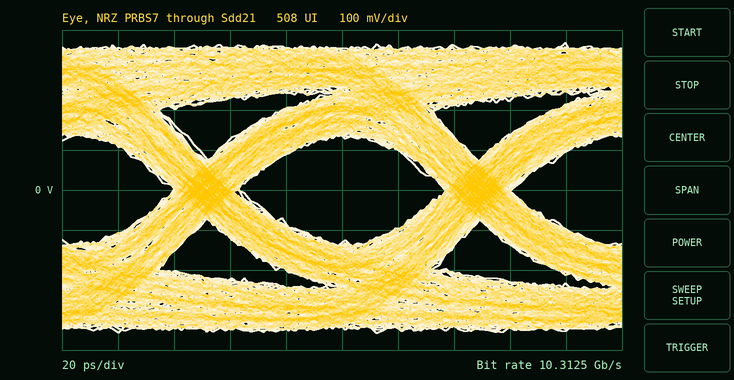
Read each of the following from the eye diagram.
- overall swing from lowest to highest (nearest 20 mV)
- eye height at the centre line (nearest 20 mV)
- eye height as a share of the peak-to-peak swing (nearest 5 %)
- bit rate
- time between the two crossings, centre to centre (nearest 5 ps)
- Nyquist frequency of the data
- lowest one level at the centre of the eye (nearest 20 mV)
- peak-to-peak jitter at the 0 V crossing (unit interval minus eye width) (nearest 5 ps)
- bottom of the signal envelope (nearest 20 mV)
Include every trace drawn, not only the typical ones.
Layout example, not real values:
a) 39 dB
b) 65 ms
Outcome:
a) 720 mV
b) 260 mV
c) 35 %
d) 10.3125 Gb/s
e) 95 ps
f) 5.15625 GHz
g) 140 mV
h) 25 ps
i) -360 mV
